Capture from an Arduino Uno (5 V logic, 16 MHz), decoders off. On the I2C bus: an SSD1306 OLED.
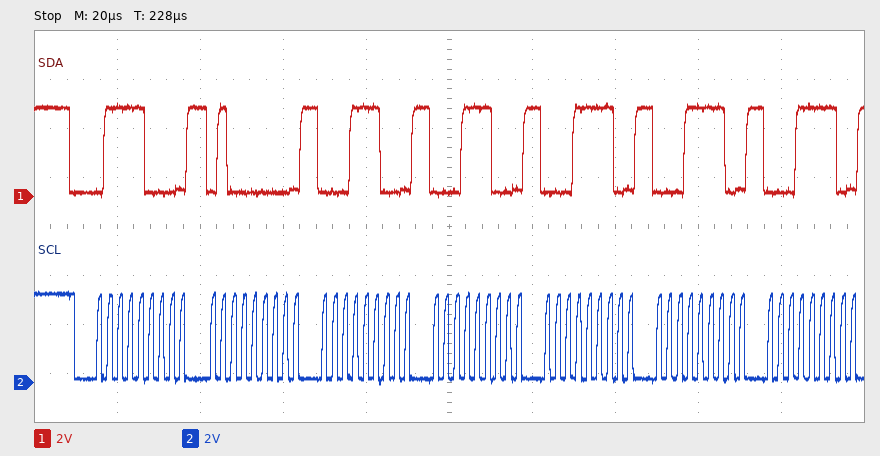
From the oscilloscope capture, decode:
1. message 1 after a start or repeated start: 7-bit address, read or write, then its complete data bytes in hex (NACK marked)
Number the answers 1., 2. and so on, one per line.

1. 0x3C write: 40 1C 1C 1E 1E 1E
